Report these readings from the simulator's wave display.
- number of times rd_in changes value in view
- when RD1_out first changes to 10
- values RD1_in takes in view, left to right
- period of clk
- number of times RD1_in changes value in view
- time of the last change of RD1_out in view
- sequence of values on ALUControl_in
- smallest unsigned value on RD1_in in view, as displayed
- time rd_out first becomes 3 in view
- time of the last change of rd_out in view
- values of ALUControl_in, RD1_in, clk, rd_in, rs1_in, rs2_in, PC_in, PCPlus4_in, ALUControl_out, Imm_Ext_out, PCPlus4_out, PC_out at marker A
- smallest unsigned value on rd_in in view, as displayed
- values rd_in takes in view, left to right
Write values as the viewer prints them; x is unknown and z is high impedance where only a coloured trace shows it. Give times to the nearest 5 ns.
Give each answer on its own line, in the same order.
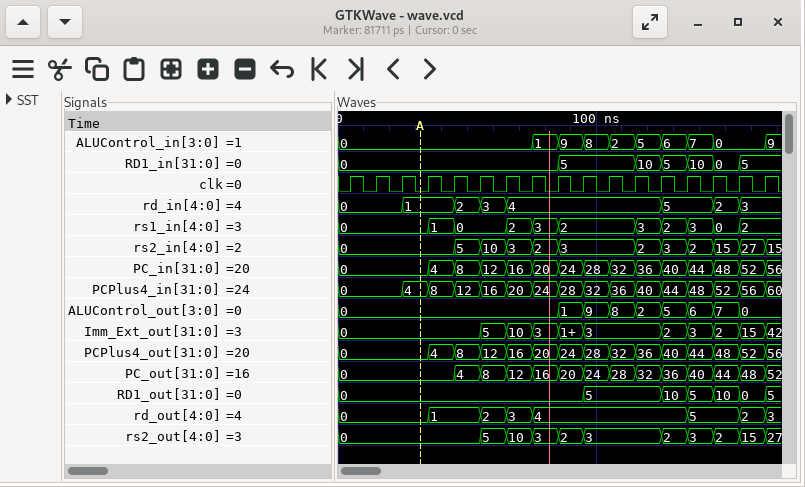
7
125 ns
0, 5, 10, 5, 10, 0, 5
10 ns
6
165 ns
0, 1, 9, 8, 2, 5, 6, 7, 0, 9
0
65 ns
165 ns
ALUControl_in=0, RD1_in=0, clk=0, rd_in=1, rs1_in=0, rs2_in=0, PC_in=0, PCPlus4_in=4, ALUControl_out=0, Imm_Ext_out=0, PCPlus4_out=0, PC_out=0
0
0, 1, 2, 3, 4, 5, 2, 3
